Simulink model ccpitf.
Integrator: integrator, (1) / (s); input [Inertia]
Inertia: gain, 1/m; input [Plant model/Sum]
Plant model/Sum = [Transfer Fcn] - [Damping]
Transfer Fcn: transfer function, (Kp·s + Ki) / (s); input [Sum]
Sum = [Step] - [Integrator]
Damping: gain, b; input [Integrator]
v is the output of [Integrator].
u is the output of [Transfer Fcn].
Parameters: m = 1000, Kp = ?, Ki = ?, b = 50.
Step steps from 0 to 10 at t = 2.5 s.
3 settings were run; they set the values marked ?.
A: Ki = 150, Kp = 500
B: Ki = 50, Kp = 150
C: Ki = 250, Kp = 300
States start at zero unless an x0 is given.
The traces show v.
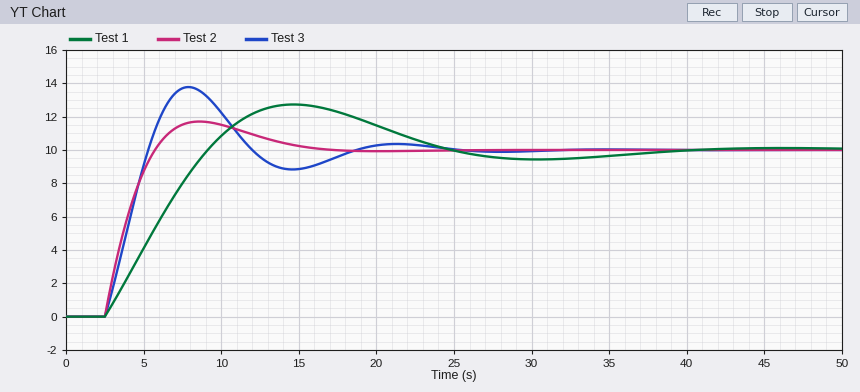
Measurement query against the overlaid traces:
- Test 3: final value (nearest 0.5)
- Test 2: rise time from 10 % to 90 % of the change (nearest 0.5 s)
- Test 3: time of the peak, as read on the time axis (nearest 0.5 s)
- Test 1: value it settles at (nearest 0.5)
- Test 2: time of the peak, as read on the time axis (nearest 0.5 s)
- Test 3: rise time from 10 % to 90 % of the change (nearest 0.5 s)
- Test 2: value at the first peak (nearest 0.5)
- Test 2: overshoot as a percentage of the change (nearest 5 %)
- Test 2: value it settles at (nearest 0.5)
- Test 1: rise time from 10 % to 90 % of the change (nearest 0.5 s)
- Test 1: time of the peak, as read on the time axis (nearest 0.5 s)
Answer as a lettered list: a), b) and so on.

a) 10.0
b) 2.5 s
c) 8.0 s
d) 10.0
e) 8.5 s
f) 2.0 s
g) 11.5
h) 15 %
i) 10.0
j) 5.0 s
k) 14.5 s
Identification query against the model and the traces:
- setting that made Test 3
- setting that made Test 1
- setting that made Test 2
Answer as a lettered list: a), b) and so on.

a) C
b) B
c) A
